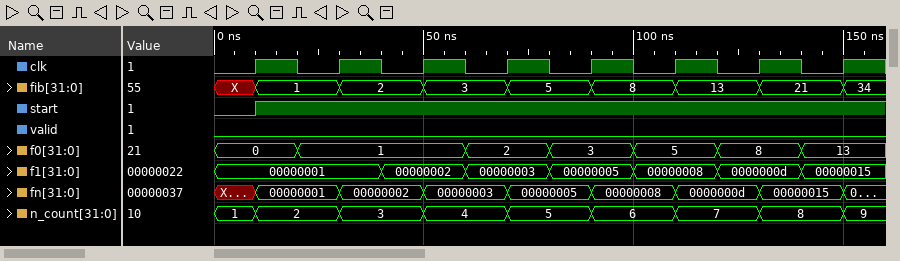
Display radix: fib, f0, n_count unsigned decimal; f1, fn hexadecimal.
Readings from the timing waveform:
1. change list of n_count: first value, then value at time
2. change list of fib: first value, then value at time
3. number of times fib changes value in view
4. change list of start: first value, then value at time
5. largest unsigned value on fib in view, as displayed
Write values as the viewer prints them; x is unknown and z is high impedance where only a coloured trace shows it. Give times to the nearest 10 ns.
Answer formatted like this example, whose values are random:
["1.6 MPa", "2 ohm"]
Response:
["1, 2 at 10 ns, 3 at 30 ns, 4 at 50 ns, 5 at 70 ns, 6 at 90 ns, 7 at 110 ns, 8 at 130 ns, 9 at 150 ns", "X, 1 at 10 ns, 2 at 30 ns, 3 at 50 ns, 5 at 70 ns, 8 at 90 ns, 13 at 110 ns, 21 at 130 ns, 34 at 150 ns", "8", "0, 1 at 10 ns", "34"]
